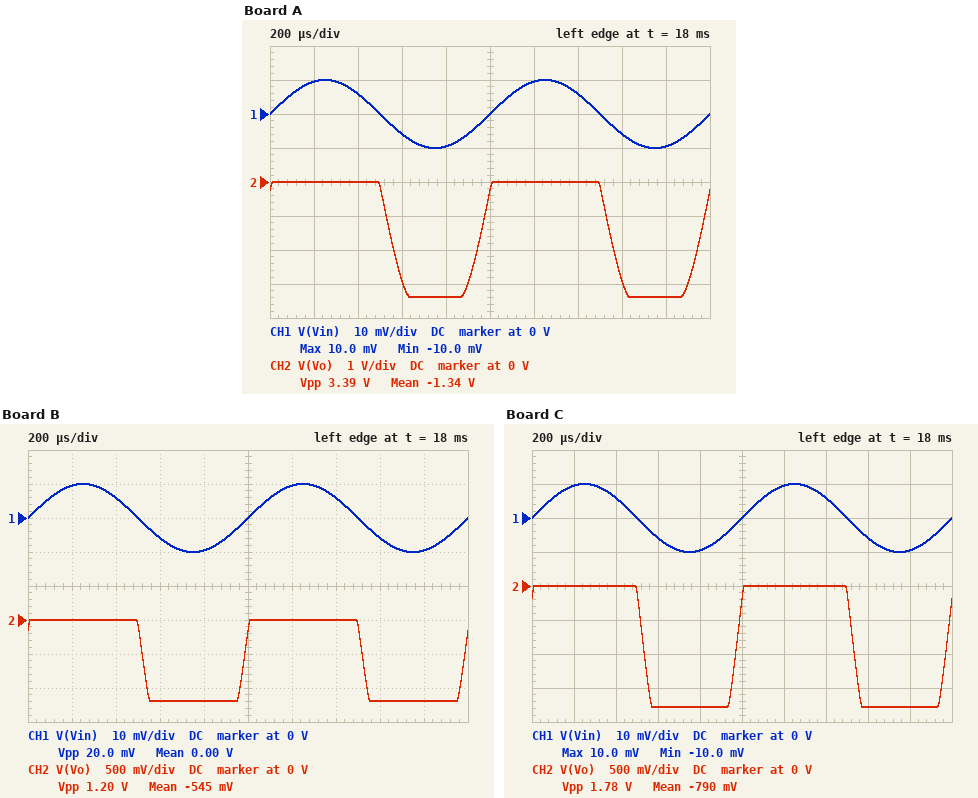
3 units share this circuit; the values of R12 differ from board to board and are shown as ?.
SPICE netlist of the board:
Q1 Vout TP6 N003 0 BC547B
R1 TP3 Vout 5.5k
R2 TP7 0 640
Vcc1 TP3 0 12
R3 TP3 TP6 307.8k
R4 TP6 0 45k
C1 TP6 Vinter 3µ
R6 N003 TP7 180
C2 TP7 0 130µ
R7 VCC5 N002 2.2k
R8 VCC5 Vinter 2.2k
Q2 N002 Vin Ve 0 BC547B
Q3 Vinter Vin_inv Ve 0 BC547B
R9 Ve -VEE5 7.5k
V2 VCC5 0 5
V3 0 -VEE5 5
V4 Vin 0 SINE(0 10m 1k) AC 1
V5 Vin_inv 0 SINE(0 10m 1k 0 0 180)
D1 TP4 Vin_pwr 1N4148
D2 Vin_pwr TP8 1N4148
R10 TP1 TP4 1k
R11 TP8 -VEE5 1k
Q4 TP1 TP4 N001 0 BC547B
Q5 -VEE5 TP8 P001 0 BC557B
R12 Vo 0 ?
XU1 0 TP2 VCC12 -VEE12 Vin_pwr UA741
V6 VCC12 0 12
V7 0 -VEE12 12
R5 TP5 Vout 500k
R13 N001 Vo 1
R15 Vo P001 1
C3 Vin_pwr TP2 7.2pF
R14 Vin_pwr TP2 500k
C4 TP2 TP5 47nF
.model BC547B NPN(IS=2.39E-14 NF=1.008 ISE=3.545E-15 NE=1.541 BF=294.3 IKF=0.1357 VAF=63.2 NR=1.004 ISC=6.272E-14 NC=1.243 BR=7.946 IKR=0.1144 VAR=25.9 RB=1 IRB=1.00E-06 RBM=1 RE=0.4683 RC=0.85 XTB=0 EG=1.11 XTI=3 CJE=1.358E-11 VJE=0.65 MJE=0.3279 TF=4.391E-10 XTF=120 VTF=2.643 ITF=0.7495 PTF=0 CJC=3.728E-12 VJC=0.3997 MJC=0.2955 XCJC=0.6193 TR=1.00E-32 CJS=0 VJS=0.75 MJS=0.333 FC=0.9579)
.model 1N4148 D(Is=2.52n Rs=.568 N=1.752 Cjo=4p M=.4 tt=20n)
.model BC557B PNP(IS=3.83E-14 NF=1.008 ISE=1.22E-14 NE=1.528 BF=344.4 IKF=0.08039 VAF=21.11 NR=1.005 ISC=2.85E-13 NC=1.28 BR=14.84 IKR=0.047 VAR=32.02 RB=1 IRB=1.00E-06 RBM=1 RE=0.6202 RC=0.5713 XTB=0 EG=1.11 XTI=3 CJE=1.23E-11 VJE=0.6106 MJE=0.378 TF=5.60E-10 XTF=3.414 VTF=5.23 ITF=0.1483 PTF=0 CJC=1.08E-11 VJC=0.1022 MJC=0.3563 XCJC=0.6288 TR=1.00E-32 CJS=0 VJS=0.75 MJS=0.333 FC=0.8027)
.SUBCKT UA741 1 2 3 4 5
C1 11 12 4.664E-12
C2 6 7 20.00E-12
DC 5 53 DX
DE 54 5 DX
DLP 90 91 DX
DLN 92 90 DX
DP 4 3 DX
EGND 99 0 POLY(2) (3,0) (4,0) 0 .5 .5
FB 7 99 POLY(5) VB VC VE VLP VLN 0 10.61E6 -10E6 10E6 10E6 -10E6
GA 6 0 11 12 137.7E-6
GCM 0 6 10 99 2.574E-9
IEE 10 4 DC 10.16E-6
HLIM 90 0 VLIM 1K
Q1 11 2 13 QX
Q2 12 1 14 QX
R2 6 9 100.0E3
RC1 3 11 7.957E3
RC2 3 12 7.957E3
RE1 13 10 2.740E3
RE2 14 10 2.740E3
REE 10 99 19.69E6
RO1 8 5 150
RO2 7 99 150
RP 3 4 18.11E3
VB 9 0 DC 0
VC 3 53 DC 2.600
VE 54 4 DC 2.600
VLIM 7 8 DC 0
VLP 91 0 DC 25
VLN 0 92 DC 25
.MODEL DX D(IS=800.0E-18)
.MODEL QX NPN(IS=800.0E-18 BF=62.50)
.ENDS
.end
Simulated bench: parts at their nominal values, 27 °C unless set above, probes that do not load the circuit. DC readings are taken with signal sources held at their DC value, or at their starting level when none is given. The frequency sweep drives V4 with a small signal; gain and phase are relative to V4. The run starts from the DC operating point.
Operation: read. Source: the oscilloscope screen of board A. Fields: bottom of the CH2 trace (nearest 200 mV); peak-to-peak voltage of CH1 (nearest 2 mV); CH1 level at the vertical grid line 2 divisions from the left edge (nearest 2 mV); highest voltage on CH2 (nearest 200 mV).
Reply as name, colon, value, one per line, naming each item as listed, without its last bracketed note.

bottom of the CH2 trace: -3.4 V
peak-to-peak voltage of CH1: 20 mV
CH1 level at the vertical grid line 2 divisions from the left edge: 6 mV
highest voltage on CH2: 0 V
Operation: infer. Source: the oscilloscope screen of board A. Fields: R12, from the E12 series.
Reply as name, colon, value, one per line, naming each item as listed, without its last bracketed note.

R12, from the E12 series: 33 Ω
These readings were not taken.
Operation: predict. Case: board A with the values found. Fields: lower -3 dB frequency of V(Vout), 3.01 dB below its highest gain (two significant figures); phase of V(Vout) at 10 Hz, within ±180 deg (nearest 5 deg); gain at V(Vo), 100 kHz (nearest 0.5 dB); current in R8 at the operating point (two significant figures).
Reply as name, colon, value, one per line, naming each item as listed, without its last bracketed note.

lower -3 dB frequency of V(Vout), 3.01 dB below its highest gain: 7.9 Hz
phase of V(Vout) at 10 Hz, within ±180 deg: -145 deg
gain at V(Vo), 100 kHz: 31.5 dB
current in R8 at the operating point: 290 µA
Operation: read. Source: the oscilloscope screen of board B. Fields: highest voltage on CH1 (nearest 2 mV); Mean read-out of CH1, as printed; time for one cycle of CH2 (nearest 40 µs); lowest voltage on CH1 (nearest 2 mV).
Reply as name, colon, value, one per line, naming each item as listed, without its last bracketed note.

highest voltage on CH1: 10 mV
Mean read-out of CH1, as printed: 0.00 V
time for one cycle of CH2: 1.00 ms
lowest voltage on CH1: -10 mV
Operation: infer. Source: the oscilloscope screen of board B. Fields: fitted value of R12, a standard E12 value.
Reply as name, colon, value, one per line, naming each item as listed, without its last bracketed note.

fitted value of R12, a standard E12 value: 4.7 Ω
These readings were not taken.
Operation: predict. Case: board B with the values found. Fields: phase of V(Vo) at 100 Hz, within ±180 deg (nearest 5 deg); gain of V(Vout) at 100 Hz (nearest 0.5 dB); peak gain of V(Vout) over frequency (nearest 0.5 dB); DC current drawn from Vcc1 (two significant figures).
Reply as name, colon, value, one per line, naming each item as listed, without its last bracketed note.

phase of V(Vo) at 100 Hz, within ±180 deg: 10 deg
gain of V(Vout) at 100 Hz: 49.0 dB
peak gain of V(Vout) over frequency: 49.0 dB
DC current drawn from Vcc1: 980 µA
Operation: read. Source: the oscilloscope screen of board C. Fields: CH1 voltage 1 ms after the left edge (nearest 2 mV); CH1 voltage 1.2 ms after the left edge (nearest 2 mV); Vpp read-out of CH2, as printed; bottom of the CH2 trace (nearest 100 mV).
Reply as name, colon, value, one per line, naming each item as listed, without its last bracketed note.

CH1 voltage 1 ms after the left edge: 0 V
CH1 voltage 1.2 ms after the left edge: 10 mV
Vpp read-out of CH2, as printed: 1.78 V
bottom of the CH2 trace: -1.8 V
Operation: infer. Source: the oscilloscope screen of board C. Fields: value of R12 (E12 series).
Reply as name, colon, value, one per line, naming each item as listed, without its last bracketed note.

value of R12: 8.2 Ω
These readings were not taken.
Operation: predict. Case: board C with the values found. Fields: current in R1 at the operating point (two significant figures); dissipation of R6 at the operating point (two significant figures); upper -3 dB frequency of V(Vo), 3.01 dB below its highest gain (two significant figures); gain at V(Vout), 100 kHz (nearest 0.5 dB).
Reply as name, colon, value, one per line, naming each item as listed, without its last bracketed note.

current in R1 at the operating point: 940 µA
dissipation of R6 at the operating point: 160 µW
upper -3 dB frequency of V(Vo), 3.01 dB below its highest gain: 41 kHz
gain at V(Vout), 100 kHz: 49.0 dB
